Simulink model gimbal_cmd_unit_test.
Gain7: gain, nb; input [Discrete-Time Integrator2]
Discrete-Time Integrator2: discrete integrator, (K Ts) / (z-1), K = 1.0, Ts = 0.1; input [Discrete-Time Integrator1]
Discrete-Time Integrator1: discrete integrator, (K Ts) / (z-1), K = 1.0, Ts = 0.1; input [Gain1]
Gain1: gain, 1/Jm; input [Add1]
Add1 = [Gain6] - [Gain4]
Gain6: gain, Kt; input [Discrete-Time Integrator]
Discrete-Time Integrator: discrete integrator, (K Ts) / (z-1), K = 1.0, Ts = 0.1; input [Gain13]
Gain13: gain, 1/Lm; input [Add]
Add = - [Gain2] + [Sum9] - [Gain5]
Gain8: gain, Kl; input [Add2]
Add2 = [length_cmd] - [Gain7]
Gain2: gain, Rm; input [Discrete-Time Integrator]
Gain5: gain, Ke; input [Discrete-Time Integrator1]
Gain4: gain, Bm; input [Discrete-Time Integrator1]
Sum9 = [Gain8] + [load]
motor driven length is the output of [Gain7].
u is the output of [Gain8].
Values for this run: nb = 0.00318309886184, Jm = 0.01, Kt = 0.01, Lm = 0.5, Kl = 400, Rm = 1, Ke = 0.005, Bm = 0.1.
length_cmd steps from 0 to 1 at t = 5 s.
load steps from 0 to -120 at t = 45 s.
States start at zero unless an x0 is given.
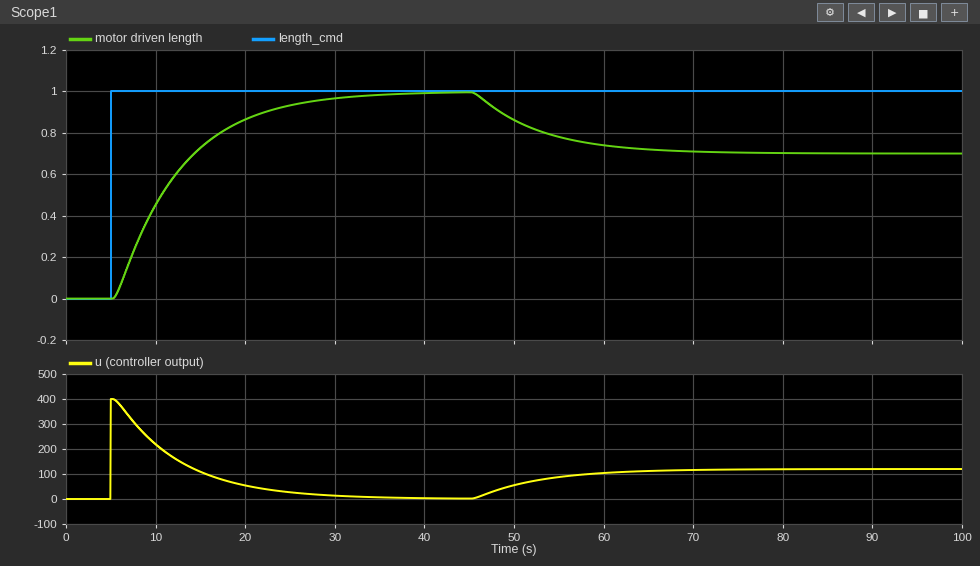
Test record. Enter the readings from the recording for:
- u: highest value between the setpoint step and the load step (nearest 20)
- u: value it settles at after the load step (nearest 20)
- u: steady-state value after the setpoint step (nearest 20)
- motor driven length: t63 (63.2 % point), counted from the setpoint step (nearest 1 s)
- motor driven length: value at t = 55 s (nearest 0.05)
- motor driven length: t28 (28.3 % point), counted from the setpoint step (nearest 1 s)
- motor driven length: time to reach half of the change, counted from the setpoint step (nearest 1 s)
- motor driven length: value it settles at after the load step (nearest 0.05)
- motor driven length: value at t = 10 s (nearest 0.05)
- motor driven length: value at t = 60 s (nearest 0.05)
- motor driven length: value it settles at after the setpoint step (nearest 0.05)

400
120
0
8 s
0.80
3 s
6 s
0.70
0.45
0.75
1.00
